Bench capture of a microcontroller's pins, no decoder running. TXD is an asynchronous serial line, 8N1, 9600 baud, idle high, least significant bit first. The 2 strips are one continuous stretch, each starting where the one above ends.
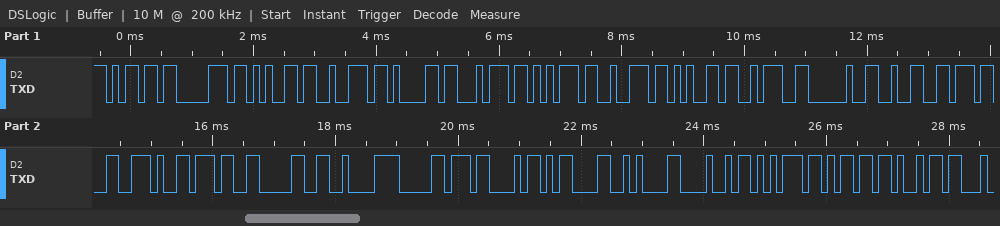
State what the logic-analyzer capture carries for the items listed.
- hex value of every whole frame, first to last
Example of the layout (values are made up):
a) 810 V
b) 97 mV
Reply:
a) 6D 70 65 72 61 74 75 72 65 3A 20 32 37 2E 37 30 C2 B0 43 0D 0A 48 75 6D 69
